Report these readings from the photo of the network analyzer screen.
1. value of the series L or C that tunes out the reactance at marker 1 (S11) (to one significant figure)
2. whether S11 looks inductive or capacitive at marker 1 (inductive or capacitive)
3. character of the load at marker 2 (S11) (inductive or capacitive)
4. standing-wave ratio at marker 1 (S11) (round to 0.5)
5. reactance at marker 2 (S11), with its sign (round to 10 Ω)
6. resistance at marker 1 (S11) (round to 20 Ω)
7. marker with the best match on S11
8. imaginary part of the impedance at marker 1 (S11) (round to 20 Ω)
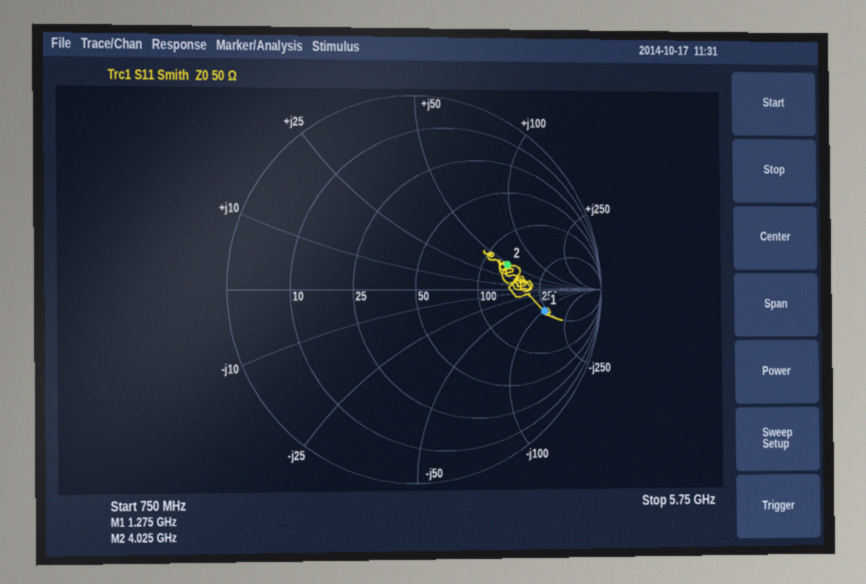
10 nH
capacitive
inductive
5.5
+50 Ω
240 Ω
marker 2
-100 Ω
